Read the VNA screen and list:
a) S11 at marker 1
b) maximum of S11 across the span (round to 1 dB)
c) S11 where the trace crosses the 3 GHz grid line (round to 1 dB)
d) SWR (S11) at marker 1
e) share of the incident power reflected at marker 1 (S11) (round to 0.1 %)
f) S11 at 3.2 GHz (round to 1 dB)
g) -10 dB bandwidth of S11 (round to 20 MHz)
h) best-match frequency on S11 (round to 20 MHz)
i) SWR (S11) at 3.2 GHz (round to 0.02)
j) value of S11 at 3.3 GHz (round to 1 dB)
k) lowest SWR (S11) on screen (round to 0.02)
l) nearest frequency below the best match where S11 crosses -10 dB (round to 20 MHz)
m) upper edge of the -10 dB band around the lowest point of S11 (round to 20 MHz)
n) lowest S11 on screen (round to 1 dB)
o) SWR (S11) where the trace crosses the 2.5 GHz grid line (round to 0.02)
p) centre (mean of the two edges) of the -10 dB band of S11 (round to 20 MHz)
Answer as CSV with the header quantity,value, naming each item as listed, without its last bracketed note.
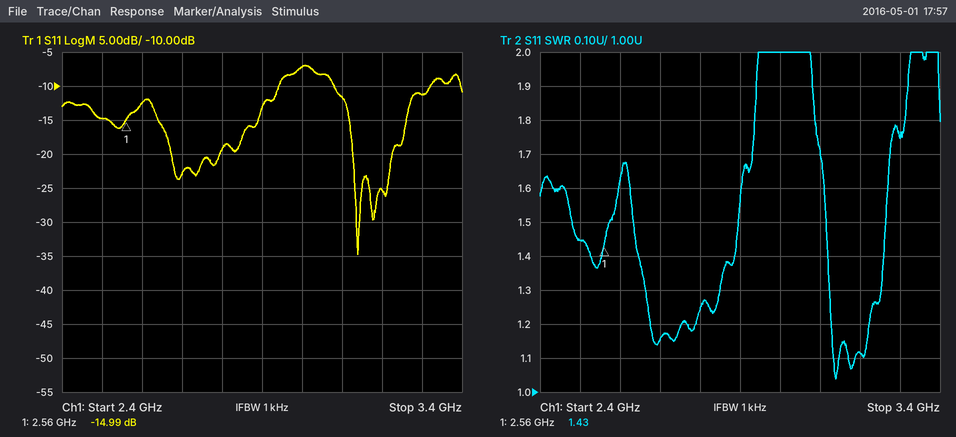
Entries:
quantity,value
S11 at marker 1,-14.99 dB
maximum of S11 across the span,-7 dB
S11 where the trace crosses the 3 GHz grid line,-7 dB
SWR (S11) at marker 1,1.43
share of the incident power reflected at marker 1 (S11),3.2 %
S11 at 3.2 GHz,-25 dB
-10 dB bandwidth of S11,240 MHz
best-match frequency on S11,3.14 GHz
SWR (S11) at 3.2 GHz,1.12
value of S11 at 3.3 GHz,-11 dB
lowest SWR (S11) on screen,1.04
nearest frequency below the best match where S11 crosses -10 dB,3.08 GHz
upper edge of the -10 dB band around the lowest point of S11,3.32 GHz
lowest S11 on screen,-35 dB
SWR (S11) where the trace crosses the 2.5 GHz grid line,1.44
centre (mean of the two edges) of the -10 dB band of S11,3.20 GHz
